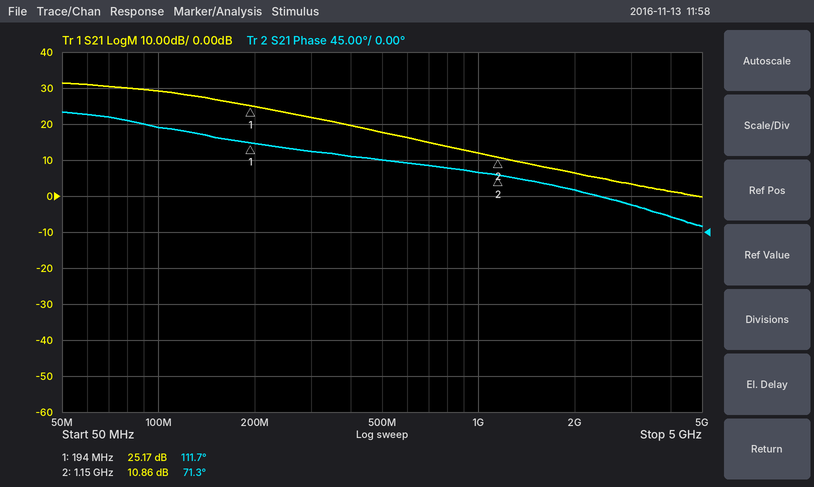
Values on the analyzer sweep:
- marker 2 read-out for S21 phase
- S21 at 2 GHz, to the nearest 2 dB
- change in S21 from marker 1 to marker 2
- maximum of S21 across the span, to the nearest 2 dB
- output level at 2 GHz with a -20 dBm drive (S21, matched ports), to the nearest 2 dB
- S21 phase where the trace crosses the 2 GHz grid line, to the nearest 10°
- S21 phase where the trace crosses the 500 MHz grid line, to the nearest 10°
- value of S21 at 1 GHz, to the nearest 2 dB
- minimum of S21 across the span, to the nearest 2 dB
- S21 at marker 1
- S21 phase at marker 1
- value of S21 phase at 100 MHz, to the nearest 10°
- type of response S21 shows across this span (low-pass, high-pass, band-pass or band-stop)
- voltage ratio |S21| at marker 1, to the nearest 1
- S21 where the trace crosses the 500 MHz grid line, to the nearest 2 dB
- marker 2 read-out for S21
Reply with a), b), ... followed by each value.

a) 71.3°
b) 6 dB
c) -14.31 dB
d) 32 dB
e) -14 dBm
f) 50°
g) 90°
h) 12 dB
i) 0 dB
j) 25.17 dB
k) 111.7°
l) 130°
m) low-pass
n) 18
o) 18 dB
p) 10.86 dB
